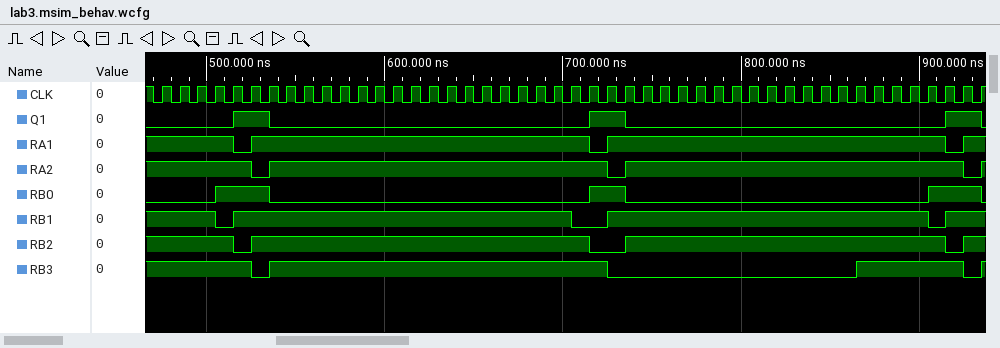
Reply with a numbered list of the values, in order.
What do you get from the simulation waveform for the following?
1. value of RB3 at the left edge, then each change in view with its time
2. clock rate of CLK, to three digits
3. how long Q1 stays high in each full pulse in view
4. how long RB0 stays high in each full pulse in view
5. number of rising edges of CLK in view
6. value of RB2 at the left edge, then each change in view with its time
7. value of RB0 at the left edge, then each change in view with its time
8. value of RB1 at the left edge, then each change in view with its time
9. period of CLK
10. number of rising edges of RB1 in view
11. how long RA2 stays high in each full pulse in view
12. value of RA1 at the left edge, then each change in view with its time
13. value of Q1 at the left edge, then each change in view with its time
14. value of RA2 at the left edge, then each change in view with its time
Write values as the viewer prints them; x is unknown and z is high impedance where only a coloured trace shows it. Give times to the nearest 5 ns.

1. 1, 0 at 525 ns, 1 at 535 ns, 0 at 725 ns, 1 at 865 ns, 0 at 925 ns, 1 at 935 ns
2. 100 MHz
3. 20 ns, 20 ns, 20 ns
4. 30 ns, 20 ns, 30 ns
5. 47
6. 1, 0 at 515 ns, 1 at 525 ns, 0 at 715 ns, 1 at 735 ns, 0 at 915 ns, 1 at 925 ns
7. 0, 1 at 505 ns, 0 at 535 ns, 1 at 715 ns, 0 at 735 ns, 1 at 905 ns, 0 at 935 ns
8. 1, 0 at 505 ns, 1 at 515 ns, 0 at 705 ns, 1 at 725 ns, 0 at 905 ns, 1 at 915 ns
9. 10 ns
10. 3
11. 190 ns, 190 ns
12. 1, 0 at 515 ns, 1 at 525 ns, 0 at 715 ns, 1 at 725 ns, 0 at 915 ns, 1 at 925 ns
13. 0, 1 at 515 ns, 0 at 535 ns, 1 at 715 ns, 0 at 735 ns, 1 at 915 ns, 0 at 935 ns
14. 1, 0 at 525 ns, 1 at 535 ns, 0 at 725 ns, 1 at 735 ns, 0 at 925 ns, 1 at 935 ns
